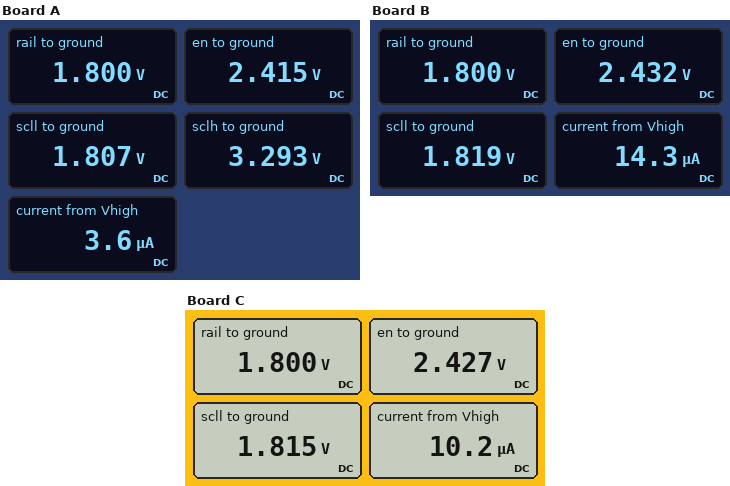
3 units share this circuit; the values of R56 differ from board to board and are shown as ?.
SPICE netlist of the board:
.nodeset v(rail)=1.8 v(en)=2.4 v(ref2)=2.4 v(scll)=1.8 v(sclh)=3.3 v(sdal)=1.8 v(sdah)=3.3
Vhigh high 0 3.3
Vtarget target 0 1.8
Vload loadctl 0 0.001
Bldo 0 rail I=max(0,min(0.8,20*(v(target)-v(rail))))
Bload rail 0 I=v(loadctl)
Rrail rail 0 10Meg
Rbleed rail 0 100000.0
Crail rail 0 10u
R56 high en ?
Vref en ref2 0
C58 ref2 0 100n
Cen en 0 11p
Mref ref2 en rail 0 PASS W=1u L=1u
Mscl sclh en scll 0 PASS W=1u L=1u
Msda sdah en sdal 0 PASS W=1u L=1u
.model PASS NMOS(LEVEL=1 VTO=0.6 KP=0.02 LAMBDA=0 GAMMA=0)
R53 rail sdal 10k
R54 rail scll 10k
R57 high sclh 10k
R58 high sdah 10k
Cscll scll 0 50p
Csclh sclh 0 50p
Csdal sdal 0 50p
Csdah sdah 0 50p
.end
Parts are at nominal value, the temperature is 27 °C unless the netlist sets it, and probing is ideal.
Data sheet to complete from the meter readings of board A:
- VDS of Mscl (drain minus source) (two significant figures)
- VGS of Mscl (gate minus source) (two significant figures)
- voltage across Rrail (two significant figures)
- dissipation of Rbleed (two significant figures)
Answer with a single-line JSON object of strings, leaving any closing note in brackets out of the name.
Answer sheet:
{"VDS of Mscl (drain minus source)": "1.5 V", "VGS of Mscl (gate minus source)": "610 mV", "voltage across Rrail": "1.8 V", "dissipation of Rbleed": "32 µW"}
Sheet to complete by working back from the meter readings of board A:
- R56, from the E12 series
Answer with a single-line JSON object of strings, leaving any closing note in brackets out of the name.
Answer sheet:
{"R56, from the E12 series": "390 kΩ"}
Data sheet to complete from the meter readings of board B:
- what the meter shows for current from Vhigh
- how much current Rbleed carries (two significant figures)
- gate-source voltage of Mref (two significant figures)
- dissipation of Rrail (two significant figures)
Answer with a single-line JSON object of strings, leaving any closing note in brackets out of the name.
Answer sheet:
{"what the meter shows for current from Vhigh": "14.3 µA", "how much current Rbleed carries": "18 µA", "gate-source voltage of Mref": "630 mV", "dissipation of Rrail": "320 nW"}
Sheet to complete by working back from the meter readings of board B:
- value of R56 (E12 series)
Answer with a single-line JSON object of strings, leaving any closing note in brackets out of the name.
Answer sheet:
{"value of R56": "82 kΩ"}
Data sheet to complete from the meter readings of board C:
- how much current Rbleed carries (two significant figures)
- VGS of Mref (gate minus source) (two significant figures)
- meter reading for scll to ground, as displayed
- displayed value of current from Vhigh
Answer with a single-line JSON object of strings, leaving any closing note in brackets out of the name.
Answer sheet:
{"how much current Rbleed carries": "18 µA", "VGS of Mref (gate minus source)": "630 mV", "meter reading for scll to ground, as displayed": "1.815 V", "displayed value of current from Vhigh": "10.2 µA"}
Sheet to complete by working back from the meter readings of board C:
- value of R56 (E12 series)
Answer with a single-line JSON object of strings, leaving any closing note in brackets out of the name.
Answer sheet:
{"value of R56": "120 kΩ"}
